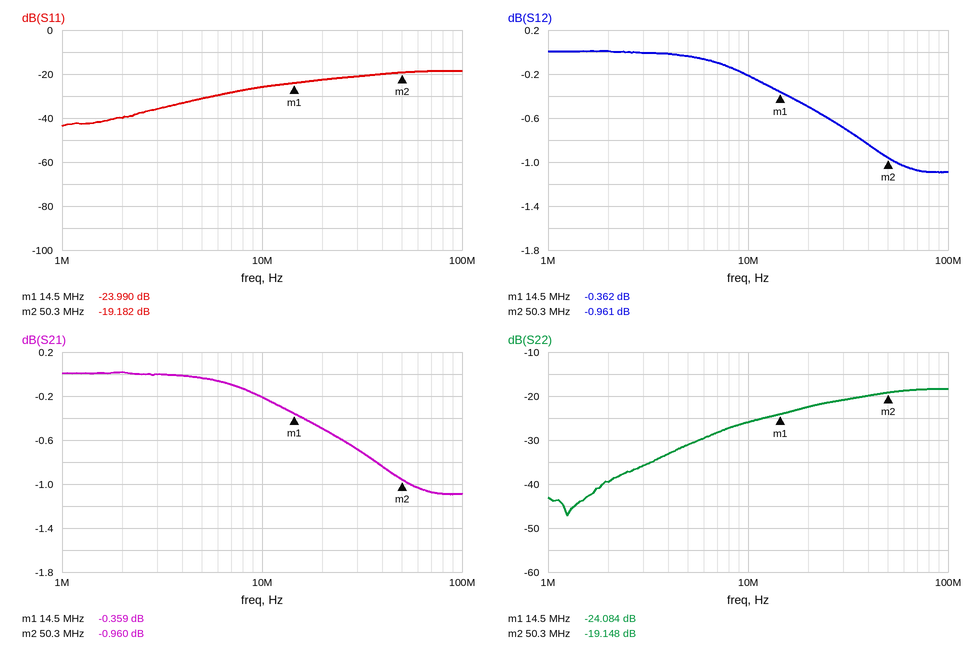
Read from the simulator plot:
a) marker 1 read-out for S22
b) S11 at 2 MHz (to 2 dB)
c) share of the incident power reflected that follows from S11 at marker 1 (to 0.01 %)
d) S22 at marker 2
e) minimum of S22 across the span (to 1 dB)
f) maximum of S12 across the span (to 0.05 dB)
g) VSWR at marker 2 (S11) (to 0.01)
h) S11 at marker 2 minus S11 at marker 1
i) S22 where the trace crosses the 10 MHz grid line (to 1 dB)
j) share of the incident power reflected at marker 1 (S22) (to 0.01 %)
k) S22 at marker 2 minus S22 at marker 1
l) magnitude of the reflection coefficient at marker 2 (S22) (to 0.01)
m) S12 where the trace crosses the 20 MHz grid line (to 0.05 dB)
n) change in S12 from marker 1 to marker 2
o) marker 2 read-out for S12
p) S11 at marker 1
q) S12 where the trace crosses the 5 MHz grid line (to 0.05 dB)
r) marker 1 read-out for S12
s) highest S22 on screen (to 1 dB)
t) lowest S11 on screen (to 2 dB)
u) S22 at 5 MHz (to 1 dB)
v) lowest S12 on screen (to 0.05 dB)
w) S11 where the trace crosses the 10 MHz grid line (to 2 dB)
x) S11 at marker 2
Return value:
-24.084 dB
-40 dB
0.40 %
-19.148 dB
-47 dB
0.00 dB
1.25
4.808 dB
-26 dB
0.39 %
4.936 dB
0.11
-0.50 dB
-0.599 dB
-0.961 dB
-23.990 dB
-0.05 dB
-0.362 dB
-18 dB
-44 dB
-31 dB
-1.10 dB
-26 dB
-19.182 dB
